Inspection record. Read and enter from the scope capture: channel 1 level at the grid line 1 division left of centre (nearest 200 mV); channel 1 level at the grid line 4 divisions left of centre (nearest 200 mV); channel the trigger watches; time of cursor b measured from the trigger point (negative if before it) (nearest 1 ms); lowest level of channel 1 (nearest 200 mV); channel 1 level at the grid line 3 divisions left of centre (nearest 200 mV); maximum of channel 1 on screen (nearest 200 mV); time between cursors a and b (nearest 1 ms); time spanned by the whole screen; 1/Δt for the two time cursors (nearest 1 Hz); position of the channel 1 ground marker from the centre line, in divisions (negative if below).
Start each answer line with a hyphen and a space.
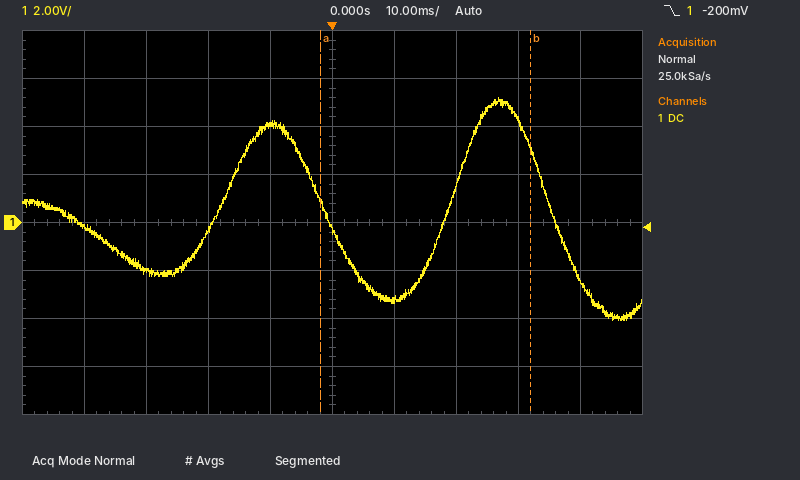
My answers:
- 4.0 V
- -200 mV
- channel 1
- +32 ms
- -4.0 V
- -2.0 V
- 5.2 V
- 34 ms
- 100 ms
- 29 Hz
- 0.0 div
